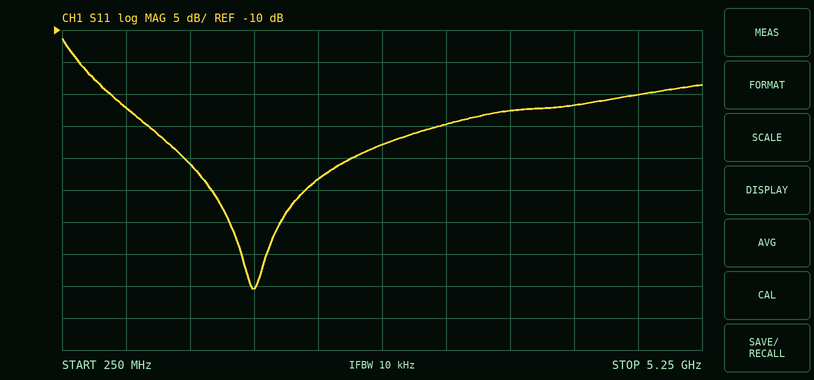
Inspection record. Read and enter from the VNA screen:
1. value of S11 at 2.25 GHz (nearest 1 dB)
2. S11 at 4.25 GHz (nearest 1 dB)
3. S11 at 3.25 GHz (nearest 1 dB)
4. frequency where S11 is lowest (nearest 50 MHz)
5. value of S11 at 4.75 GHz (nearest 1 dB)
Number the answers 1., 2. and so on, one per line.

1. -33 dB
2. -22 dB
3. -25 dB
4. 1.75 GHz
5. -20 dB
